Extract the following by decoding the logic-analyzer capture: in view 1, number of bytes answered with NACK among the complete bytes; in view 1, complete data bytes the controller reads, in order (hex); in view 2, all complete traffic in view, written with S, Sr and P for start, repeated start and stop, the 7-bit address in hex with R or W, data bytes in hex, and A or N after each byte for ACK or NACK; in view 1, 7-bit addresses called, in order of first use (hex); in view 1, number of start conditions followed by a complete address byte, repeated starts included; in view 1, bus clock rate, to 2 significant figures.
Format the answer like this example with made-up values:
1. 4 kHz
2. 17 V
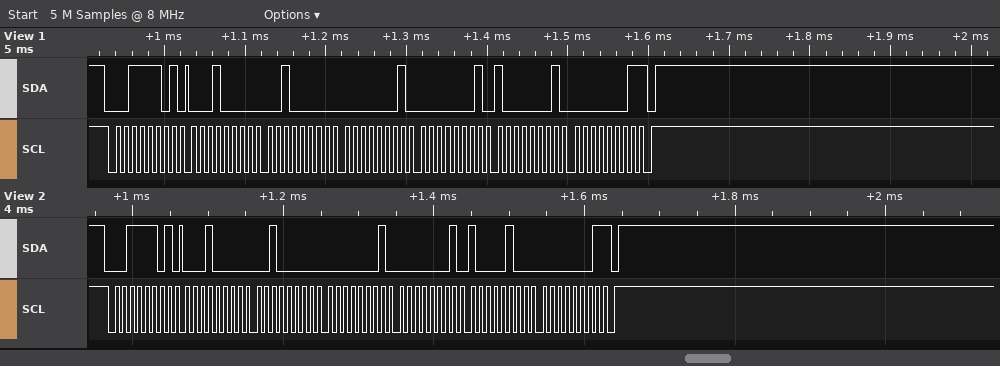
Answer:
1. 1
2. 10 20 01 01 81 01
3. S 1ER A 10 A 20 A 01 A 01 A 84 A 01 N P
4. 0x1E
5. 1
6. 100 kHz
